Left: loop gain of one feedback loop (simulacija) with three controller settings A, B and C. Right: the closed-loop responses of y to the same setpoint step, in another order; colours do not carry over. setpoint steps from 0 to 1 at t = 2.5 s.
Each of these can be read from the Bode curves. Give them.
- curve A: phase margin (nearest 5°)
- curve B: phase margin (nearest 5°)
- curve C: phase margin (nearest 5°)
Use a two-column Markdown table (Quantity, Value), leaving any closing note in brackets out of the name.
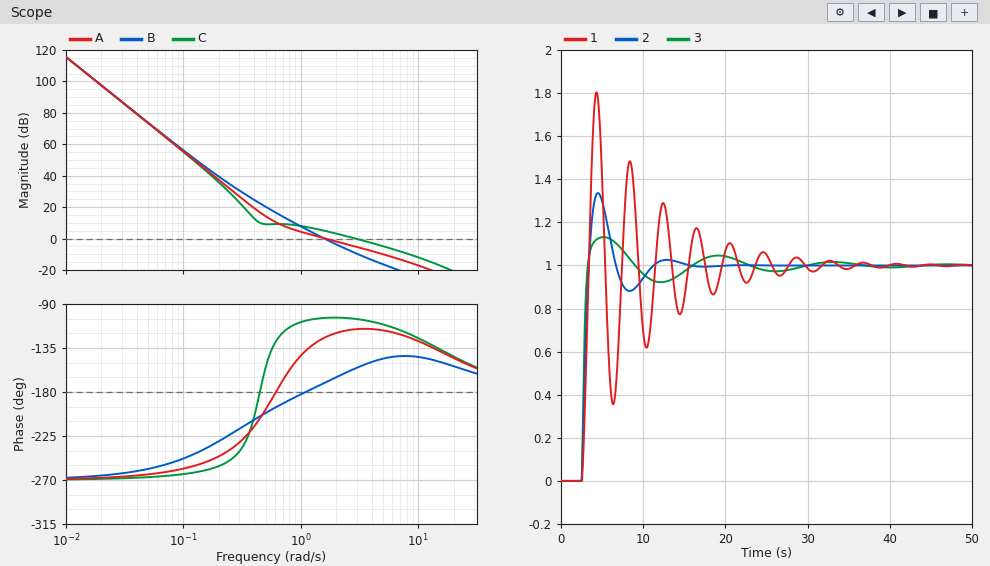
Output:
| Quantity | Value |
|---|---|
| curve A: phase margin | 55° |
| curve B: phase margin | 10° |
| curve C: phase margin | 75° |
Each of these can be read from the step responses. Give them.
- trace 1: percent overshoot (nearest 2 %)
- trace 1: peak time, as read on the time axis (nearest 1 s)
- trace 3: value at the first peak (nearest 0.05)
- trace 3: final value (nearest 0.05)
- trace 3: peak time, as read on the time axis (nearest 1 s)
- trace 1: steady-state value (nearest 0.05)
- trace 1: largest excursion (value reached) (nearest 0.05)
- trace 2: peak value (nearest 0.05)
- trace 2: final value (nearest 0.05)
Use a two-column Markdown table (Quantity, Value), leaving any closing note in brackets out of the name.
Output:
| Quantity | Value |
|---|---|
| trace 1: percent overshoot | 80 % |
| trace 1: peak time, as read on the time axis | 4 s |
| trace 3: value at the first peak | 1.15 |
| trace 3: final value | 1.00 |
| trace 3: peak time, as read on the time axis | 5 s |
| trace 1: steady-state value | 1.00 |
| trace 1: largest excursion (value reached) | 1.80 |
| trace 2: peak value | 1.35 |
| trace 2: final value | 1.00 |
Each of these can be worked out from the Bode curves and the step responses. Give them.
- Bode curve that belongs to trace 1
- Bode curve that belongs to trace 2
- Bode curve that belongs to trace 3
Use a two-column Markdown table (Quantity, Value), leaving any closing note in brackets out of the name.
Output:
| Quantity | Value |
|---|---|
| Bode curve that belongs to trace 1 | B |
| Bode curve that belongs to trace 2 | A |
| Bode curve that belongs to trace 3 | C |
